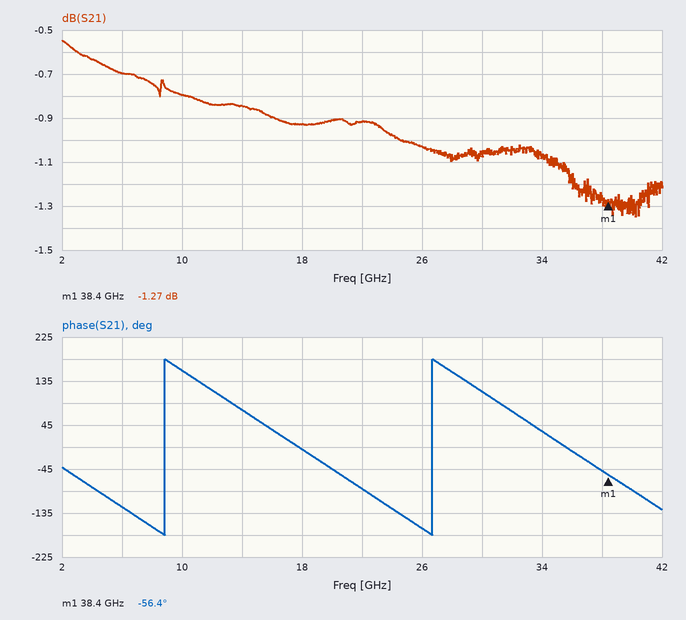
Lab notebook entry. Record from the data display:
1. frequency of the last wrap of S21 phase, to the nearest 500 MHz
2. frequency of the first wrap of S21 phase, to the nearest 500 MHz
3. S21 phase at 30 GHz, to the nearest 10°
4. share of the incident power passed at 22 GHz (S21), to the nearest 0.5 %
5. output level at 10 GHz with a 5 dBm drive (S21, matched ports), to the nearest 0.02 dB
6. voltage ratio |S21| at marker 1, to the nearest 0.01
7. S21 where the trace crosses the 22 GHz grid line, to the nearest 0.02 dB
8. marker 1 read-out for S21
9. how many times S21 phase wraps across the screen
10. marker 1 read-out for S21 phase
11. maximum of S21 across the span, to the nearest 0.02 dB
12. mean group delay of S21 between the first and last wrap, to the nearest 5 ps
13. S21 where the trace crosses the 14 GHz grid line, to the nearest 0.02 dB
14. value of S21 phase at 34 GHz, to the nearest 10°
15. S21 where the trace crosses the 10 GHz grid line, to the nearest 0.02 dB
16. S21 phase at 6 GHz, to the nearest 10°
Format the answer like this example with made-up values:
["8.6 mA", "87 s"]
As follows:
["26.5 GHz", "9.0 GHz", "110°", "81.0 %", "4.20 dBm", "0.86", "-0.92 dB", "-1.27 dB", "2", "-56.4°", "-0.54 dB", "55 ps", "-0.84 dB", "30°", "-0.80 dB", "-120°"]
